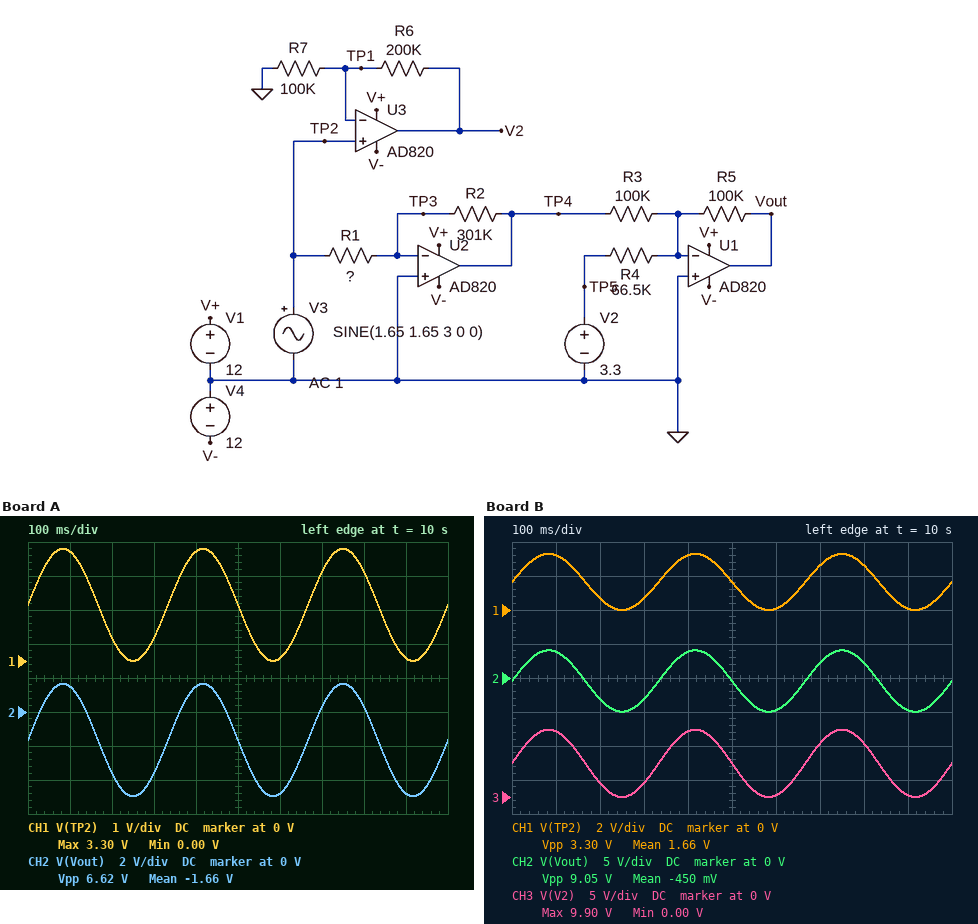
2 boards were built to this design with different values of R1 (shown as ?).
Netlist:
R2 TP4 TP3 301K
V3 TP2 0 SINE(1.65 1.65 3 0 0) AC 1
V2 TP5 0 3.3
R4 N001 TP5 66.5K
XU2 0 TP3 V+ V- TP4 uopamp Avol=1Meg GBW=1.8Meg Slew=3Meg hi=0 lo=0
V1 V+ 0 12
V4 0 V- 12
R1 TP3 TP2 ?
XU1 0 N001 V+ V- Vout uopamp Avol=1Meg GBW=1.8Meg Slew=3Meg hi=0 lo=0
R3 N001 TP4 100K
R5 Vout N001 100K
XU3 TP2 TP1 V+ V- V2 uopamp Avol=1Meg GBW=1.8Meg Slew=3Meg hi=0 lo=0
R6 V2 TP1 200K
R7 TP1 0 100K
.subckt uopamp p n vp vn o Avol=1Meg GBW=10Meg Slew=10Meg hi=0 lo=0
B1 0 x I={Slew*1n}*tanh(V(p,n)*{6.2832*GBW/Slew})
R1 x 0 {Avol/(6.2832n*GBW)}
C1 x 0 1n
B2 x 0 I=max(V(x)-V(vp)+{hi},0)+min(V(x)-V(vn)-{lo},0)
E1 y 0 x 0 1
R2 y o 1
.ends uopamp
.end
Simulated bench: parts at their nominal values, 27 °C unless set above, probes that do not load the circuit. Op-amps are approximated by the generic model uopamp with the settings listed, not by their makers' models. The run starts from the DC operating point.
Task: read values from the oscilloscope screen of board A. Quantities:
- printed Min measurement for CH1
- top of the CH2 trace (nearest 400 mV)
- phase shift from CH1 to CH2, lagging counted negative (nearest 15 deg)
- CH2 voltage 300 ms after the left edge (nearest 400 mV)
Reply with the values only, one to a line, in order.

0.00 V
1.6 V
0 deg
-3.6 V
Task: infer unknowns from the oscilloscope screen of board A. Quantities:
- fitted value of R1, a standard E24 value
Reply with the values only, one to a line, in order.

150 kΩ
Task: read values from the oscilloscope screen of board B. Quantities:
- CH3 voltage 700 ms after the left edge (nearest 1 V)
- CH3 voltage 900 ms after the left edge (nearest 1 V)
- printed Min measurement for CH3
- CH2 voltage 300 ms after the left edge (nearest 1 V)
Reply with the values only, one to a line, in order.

8 V
0 V
0.00 V
-3 V
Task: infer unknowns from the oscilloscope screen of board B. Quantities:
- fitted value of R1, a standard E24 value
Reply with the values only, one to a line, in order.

110 kΩ
